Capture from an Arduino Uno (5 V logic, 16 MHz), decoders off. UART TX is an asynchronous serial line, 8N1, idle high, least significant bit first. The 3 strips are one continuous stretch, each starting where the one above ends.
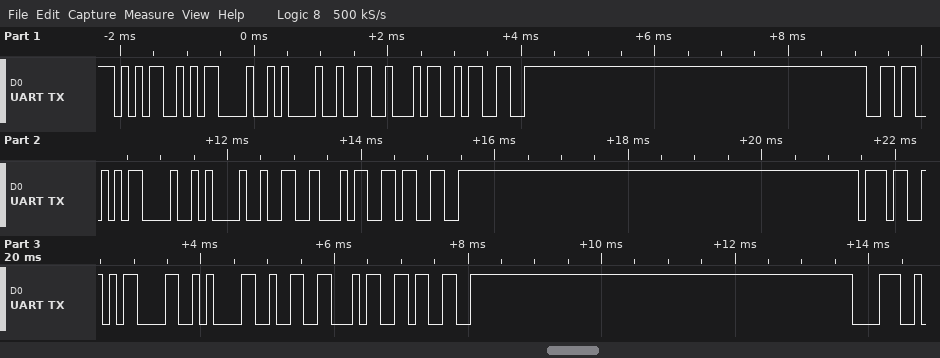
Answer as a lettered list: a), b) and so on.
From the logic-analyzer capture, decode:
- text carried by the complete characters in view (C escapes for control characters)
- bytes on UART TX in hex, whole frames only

a) "5\r\n2436\r\n2437\r\n2438"
b) 35 0D 0A 32 34 33 36 0D 0A 32 34 33 37 0D 0A 32 34 33 38
